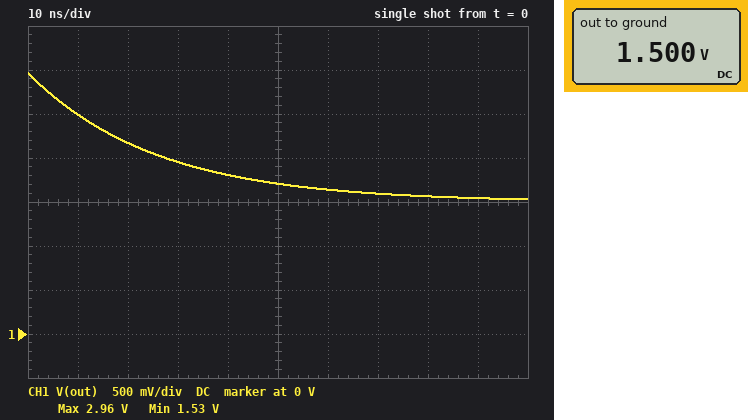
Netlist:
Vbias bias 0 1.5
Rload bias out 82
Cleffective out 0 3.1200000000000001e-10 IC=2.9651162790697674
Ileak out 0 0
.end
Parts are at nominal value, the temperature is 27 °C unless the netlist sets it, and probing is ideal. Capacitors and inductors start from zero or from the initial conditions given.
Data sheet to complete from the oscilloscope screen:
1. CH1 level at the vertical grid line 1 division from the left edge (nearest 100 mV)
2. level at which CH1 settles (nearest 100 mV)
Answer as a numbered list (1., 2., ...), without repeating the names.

1. 2.5 V
2. 1.5 V
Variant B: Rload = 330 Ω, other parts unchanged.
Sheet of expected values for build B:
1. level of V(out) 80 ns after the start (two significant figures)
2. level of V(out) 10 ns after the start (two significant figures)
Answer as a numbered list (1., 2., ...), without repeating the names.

1. 2.2 V
2. 2.8 V
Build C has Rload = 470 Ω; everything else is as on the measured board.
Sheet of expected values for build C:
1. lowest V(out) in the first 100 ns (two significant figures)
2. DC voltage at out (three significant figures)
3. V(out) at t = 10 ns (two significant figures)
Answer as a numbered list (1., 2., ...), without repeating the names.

1. 2.2 V
2. 1.50 V
3. 2.9 V
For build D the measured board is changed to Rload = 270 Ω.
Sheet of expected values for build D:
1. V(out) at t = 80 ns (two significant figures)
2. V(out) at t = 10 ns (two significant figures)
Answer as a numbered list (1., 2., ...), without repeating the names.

1. 2.1 V
2. 2.8 V
